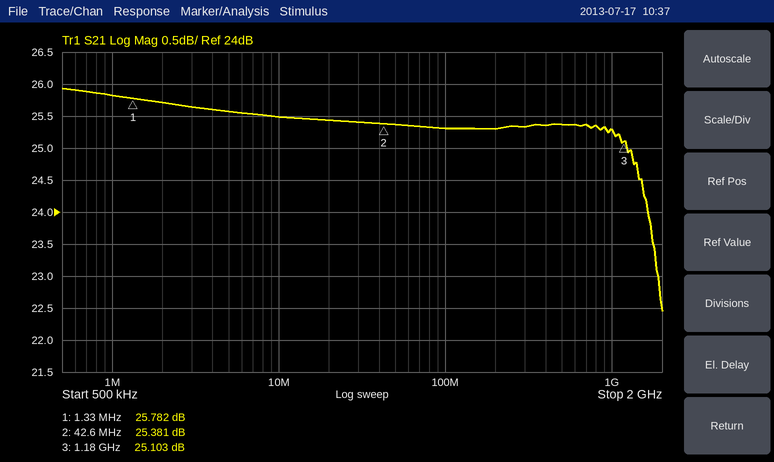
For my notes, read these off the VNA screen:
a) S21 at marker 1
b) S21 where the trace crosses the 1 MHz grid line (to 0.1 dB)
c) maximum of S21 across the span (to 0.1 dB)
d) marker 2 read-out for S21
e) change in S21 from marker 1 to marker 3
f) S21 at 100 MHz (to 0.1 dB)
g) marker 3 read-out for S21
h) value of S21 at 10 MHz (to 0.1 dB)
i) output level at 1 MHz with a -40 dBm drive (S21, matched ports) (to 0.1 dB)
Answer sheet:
25.782 dB
25.8 dB
25.9 dB
25.381 dB
-0.679 dB
25.3 dB
25.103 dB
25.5 dB
-14.2 dBm
